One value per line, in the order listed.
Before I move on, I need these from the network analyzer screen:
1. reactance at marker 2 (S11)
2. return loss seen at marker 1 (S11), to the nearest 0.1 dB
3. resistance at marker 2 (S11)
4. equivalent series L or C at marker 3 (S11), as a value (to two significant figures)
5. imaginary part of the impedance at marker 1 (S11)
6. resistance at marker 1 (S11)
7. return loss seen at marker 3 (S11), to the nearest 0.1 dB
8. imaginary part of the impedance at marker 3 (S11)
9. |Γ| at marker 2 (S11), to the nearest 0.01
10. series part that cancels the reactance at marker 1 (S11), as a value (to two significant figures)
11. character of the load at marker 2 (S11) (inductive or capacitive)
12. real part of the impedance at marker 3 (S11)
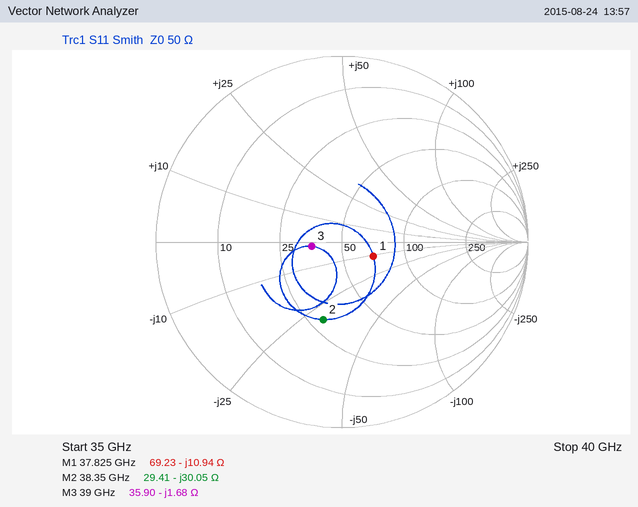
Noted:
-30.05 Ω
14.7 dB
29.41 Ω
2.4 pF
-10.94 Ω
69.23 Ω
15.6 dB
-1.68 Ω
0.43
46 pH
capacitive
35.90 Ω
